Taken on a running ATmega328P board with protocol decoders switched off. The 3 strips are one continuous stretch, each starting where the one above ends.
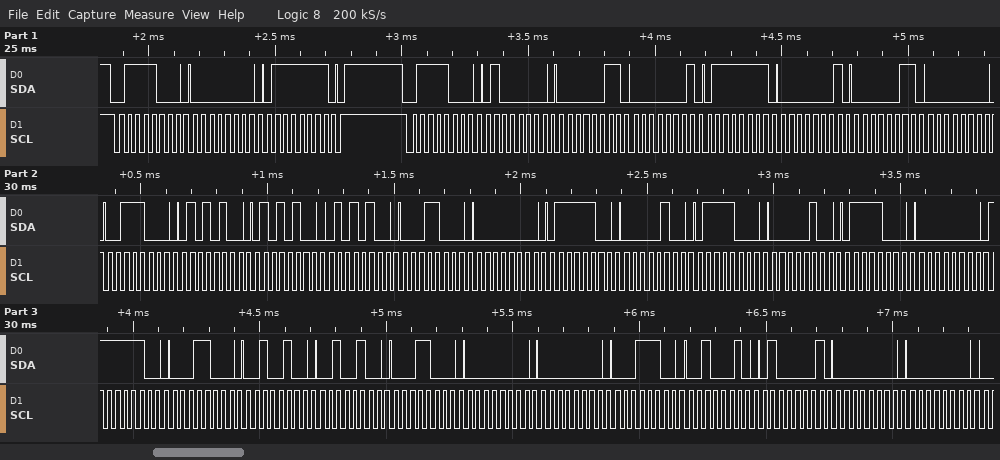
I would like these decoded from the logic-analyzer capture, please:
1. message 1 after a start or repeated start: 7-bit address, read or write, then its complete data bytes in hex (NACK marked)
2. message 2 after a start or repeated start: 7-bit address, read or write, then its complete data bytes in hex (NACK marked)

0x3C write: 00 7F
0x3C write: 40 03 01 7F 01 03 00 38 54 54 54 18 00 7C 04 78 04 78 00 FC 18 24 24 18 00 00 1C 22 41 00 00
